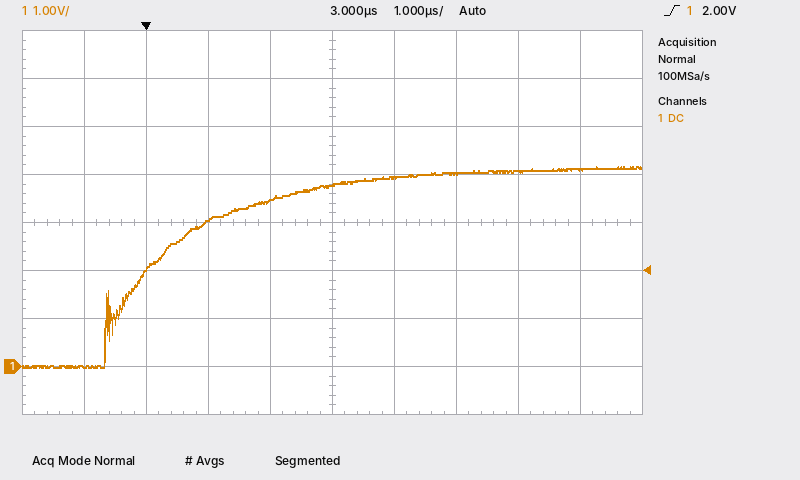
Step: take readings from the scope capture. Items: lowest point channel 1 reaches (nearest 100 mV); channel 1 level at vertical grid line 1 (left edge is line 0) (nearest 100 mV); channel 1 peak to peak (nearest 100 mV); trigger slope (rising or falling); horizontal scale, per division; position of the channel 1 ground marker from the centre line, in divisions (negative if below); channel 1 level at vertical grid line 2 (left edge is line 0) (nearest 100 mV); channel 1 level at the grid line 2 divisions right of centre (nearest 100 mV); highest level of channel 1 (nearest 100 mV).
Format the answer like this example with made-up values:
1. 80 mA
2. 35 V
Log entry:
1. 0.0 V
2. 0.0 V
3. 4.2 V
4. rising
5. 1 µs
6. -3.0 div
7. 2.0 V
8. 4.0 V
9. 4.2 V
